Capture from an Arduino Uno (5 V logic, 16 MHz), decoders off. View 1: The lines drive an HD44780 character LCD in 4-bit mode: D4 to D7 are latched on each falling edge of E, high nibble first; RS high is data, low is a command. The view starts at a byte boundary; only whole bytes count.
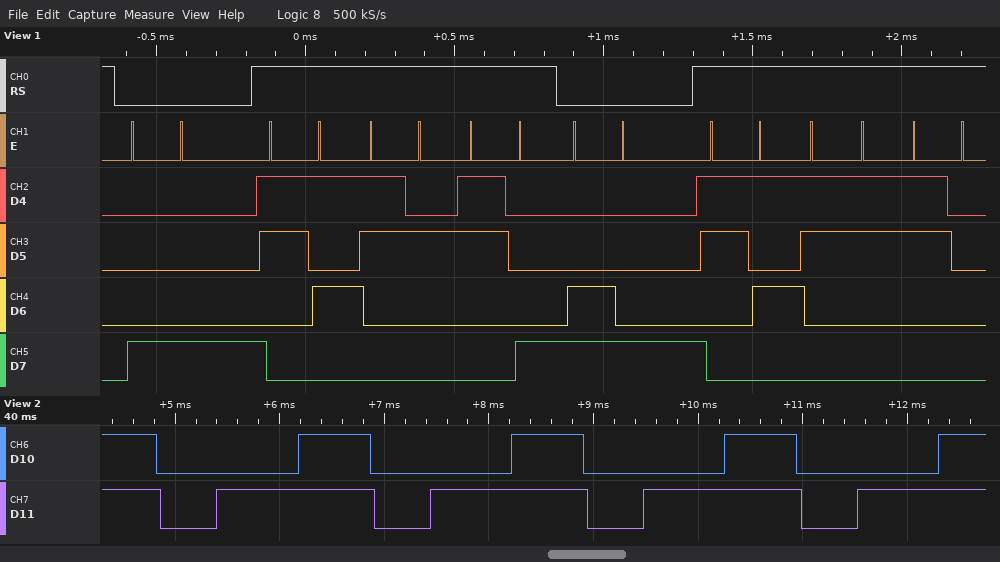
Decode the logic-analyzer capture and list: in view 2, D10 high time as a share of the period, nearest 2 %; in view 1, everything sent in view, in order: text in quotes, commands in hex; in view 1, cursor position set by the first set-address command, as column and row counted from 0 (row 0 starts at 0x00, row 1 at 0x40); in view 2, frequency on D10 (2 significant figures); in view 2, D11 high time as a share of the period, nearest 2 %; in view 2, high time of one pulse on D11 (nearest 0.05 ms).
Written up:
34 %
0x88 "528" 0xC8 "530"
column 8, row 0
490 Hz
74 %
1.50 ms
